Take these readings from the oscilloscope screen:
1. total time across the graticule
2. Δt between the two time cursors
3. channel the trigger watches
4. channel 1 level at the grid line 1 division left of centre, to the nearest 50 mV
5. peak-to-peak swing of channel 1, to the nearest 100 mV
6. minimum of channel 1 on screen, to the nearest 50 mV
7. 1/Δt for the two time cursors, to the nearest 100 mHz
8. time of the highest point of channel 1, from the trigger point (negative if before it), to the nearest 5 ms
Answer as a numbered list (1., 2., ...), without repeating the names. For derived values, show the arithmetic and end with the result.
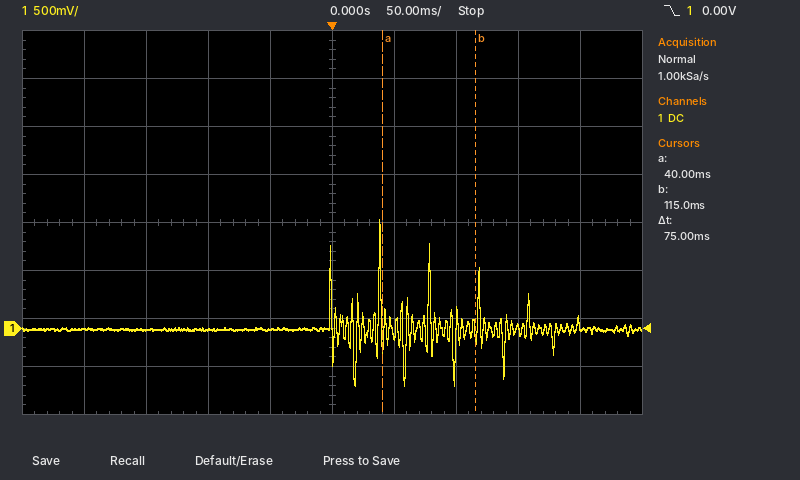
1. 500 ms
2. 75 ms
3. channel 1
4. 0 mV
5. 1.70 V
6. -600 mV
7. 1 / 75 ms ≈ 13.3 Hz
8. +40 ms
